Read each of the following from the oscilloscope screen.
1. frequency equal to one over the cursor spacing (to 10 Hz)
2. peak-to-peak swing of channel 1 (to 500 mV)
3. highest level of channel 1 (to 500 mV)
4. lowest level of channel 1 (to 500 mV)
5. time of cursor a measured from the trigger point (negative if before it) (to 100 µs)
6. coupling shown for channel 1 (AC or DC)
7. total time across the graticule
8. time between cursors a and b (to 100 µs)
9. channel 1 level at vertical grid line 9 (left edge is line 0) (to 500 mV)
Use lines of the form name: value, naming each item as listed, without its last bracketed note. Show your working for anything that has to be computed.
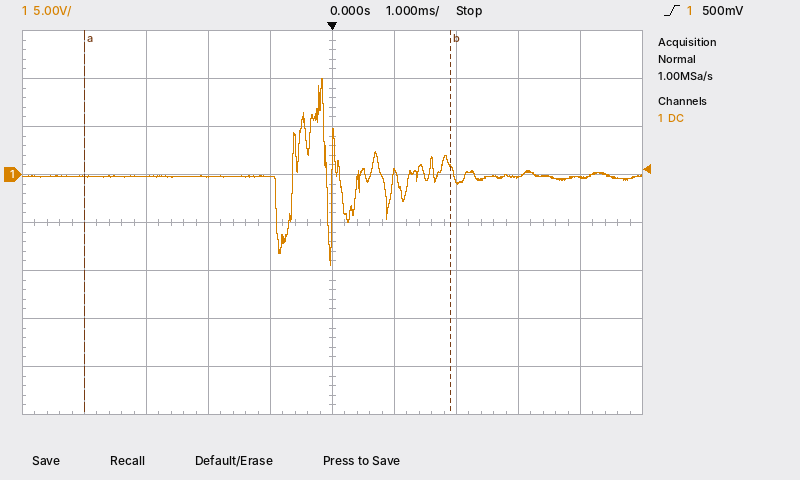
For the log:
frequency equal to one over the cursor spacing: 1 / 5.9 ms ≈ 170 Hz
peak-to-peak swing of channel 1: 10.0 V − (-9.5 V) = 19.5 V
highest level of channel 1: 10.0 V
lowest level of channel 1: -9.5 V
time of cursor a measured from the trigger point (negative if before it): -4.0 ms
coupling shown for channel 1: DC
total time across the graticule: 10 ms
time between cursors a and b: 5.9 ms
channel 1 level at vertical grid line 9 (left edge is line 0): -500 mV
